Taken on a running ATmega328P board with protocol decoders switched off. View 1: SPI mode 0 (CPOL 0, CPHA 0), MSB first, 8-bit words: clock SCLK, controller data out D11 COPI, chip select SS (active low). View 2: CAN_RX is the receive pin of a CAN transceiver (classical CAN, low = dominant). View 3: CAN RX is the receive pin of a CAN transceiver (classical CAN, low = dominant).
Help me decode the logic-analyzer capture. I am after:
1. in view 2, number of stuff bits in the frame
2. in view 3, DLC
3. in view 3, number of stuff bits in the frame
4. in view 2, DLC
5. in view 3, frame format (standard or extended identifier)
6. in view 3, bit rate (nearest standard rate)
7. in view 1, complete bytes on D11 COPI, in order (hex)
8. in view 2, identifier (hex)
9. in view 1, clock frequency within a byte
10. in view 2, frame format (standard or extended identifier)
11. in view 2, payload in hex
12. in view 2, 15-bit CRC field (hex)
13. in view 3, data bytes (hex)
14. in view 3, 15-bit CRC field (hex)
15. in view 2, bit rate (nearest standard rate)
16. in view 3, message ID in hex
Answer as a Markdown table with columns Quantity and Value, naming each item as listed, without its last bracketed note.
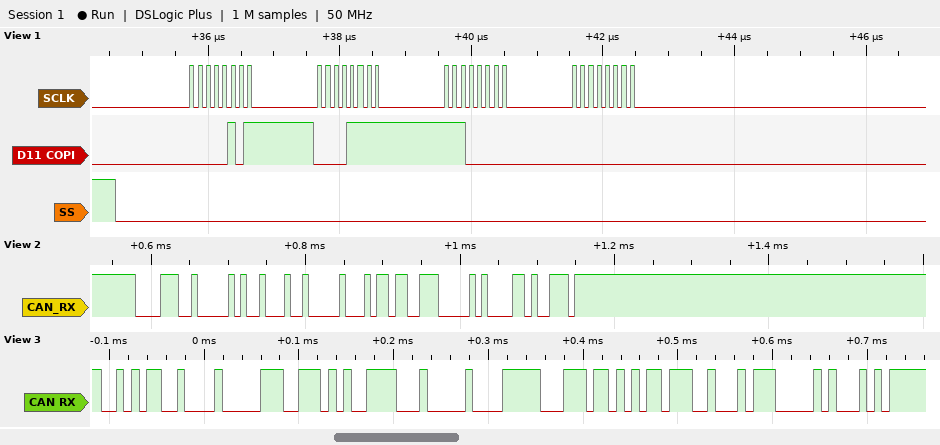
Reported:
| Quantity | Value |
|---|---|
| in view 2, number of stuff bits in the frame | 3 |
| in view 3, DLC | 8 |
| in view 3, number of stuff bits in the frame | 4 |
| in view 2, DLC | 4 |
| in view 3, frame format | standard |
| in view 3, bit rate | 125 kbit/s |
| in view 1, complete bytes on D11 COPI, in order | 05 0F E0 00 |
| in view 2, identifier | 0x0E4 |
| in view 1, clock frequency within a byte | 8 MHz |
| in view 2, frame format | standard |
| in view 2, payload in hex | 89 00 B6 70 |
| in view 2, 15-bit CRC field | 0x10D3 |
| in view 3, data bytes | 33 A9 E2 00 F9 DA B7 22 |
| in view 3, 15-bit CRC field | 0x7022 |
| in view 2, bit rate | 125 kbit/s |
| in view 3, message ID in hex | 0x2B2 |
